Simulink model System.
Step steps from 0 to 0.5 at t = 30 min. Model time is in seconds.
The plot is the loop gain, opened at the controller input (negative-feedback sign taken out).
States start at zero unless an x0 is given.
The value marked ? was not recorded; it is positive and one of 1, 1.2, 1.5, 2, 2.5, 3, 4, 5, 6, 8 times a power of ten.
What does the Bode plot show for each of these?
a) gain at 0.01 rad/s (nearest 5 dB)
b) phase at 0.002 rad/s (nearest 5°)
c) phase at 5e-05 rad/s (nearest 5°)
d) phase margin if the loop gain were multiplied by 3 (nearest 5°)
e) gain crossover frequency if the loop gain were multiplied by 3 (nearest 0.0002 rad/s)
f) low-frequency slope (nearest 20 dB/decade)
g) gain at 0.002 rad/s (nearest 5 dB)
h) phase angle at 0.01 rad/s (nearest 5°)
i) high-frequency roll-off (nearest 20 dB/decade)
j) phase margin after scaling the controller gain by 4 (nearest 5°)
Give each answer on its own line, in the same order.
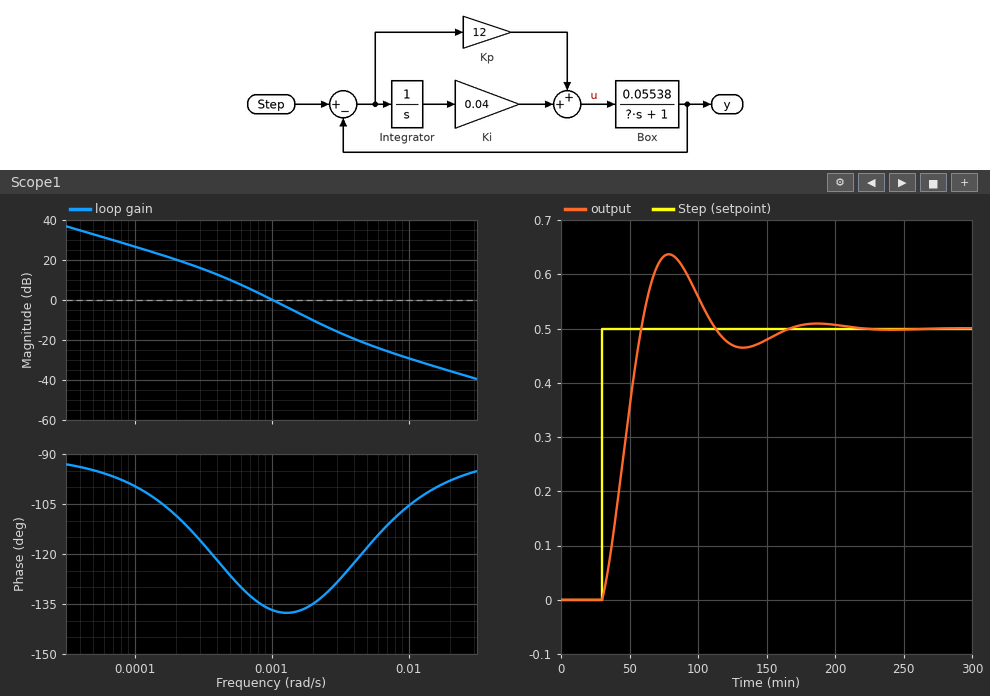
-30 dB
-135°
-95°
45°
0.0020 rad/s
-20 dB/decade
-10 dB
-105°
-20 dB/decade
45°
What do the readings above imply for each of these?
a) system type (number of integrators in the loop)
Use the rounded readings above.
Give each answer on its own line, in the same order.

1
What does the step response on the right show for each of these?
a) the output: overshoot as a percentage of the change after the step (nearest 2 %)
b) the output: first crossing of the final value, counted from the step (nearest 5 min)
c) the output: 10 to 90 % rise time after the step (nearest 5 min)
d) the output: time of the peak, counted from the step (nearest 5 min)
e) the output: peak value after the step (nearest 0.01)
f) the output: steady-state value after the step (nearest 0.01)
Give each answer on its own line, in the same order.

28 %
30 min
20 min
50 min
0.64
0.50
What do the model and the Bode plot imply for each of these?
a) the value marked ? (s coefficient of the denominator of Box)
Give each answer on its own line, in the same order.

2000
